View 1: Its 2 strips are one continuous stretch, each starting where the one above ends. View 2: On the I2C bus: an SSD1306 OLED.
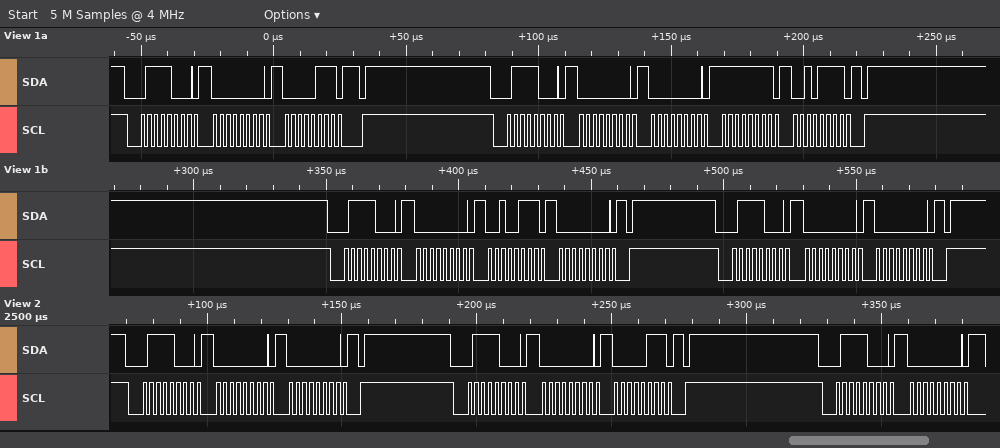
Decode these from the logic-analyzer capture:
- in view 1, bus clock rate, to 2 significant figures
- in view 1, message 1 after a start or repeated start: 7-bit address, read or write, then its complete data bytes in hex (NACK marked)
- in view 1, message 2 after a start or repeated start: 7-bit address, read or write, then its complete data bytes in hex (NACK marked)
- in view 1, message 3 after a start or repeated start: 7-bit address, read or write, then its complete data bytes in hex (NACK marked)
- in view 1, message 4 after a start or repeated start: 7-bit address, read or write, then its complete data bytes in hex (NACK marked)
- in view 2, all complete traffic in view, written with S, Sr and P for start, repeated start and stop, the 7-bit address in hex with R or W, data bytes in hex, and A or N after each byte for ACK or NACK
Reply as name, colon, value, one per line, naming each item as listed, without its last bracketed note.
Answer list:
in view 1, bus clock rate, to 2 significant figures: 400 kHz
in view 1, message 1 after a start or repeated start: 7-bit address, read or write, then its complete data bytes in hex: 0x3C write: 00 07
in view 1, message 2 after a start or repeated start: 7-bit address, read or write, then its complete data bytes in hex: 0x3C write: 00 00 FF 2F
in view 1, message 3 after a start or repeated start: 7-bit address, read or write, then its complete data bytes in hex: 0x3C write: 00 27 00
in view 1, message 4 after a start or repeated start: 7-bit address, read or write, then its complete data bytes in hex: 0x3C write: 00 00
in view 2, all complete traffic in view, written with S, Sr and P for start, repeated start and stop, the 7-bit address in hex with R or W, data bytes in hex, and A or N after each byte for ACK or NACK: S 3CW A 00 A 00 A P S 3CW A 00 A 07 A P S 3CW A 00 A
